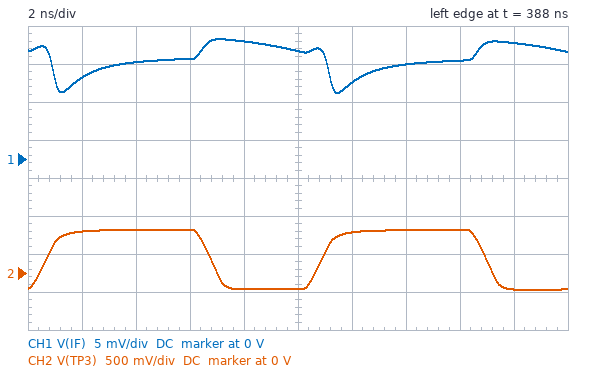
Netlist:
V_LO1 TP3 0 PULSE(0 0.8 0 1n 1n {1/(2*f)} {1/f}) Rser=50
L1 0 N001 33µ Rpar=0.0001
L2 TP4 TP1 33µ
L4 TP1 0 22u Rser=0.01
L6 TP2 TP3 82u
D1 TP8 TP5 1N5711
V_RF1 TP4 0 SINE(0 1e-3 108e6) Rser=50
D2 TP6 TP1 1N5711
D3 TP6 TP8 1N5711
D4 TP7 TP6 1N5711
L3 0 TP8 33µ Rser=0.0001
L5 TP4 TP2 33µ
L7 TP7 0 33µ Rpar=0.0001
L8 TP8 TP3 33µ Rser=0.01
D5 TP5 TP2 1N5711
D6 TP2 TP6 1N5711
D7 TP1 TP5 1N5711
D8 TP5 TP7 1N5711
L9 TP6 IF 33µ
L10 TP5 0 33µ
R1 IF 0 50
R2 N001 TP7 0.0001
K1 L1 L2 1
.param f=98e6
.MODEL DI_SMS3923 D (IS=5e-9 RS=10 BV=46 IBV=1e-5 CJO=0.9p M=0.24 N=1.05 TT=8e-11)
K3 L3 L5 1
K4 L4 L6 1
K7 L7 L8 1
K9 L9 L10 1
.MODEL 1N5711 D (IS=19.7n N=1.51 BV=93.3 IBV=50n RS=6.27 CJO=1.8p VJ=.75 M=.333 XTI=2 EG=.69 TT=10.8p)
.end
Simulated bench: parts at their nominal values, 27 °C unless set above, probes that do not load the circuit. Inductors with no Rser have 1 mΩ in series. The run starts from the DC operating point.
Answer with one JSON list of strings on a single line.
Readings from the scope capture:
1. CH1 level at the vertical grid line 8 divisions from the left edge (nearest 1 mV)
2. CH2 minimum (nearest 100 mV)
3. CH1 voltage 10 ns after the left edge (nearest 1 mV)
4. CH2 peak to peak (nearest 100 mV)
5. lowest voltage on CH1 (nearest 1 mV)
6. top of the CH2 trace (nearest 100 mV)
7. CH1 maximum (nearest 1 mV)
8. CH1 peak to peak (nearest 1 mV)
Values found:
["13 mV", "-200 mV", "14 mV", "800 mV", "9 mV", "600 mV", "16 mV", "7 mV"]
